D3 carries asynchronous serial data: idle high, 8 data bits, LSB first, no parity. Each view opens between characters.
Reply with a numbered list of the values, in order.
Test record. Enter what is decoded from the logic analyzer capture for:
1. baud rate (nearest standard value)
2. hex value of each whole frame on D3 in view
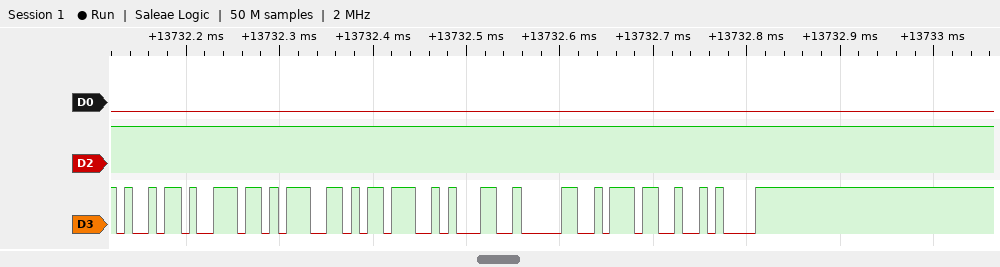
1. 115200 baud
2. 69, 6E, 67, 3B, 31, 30, 37, 0A
